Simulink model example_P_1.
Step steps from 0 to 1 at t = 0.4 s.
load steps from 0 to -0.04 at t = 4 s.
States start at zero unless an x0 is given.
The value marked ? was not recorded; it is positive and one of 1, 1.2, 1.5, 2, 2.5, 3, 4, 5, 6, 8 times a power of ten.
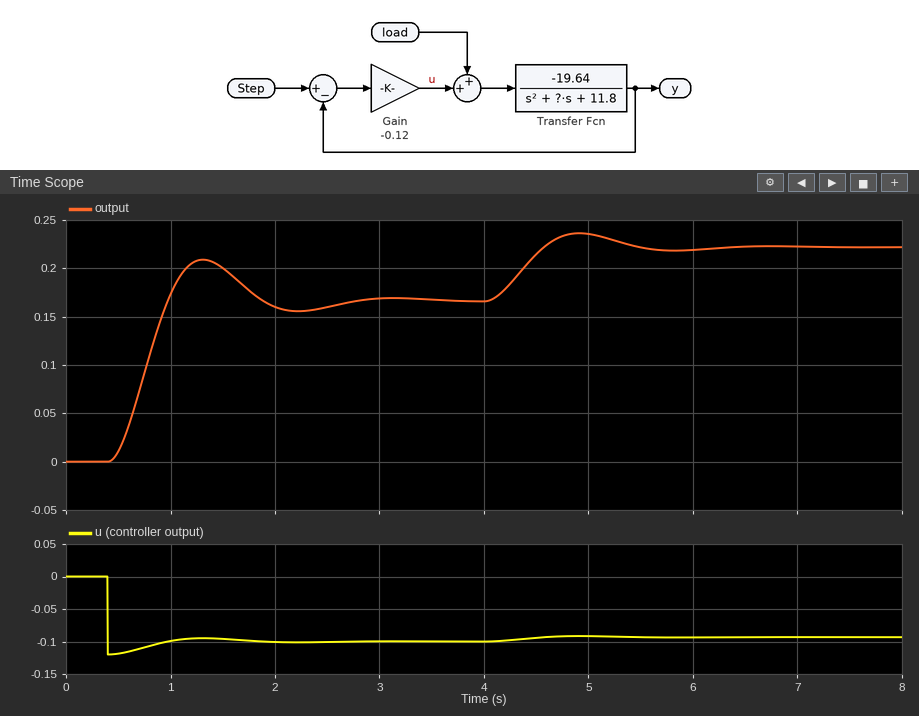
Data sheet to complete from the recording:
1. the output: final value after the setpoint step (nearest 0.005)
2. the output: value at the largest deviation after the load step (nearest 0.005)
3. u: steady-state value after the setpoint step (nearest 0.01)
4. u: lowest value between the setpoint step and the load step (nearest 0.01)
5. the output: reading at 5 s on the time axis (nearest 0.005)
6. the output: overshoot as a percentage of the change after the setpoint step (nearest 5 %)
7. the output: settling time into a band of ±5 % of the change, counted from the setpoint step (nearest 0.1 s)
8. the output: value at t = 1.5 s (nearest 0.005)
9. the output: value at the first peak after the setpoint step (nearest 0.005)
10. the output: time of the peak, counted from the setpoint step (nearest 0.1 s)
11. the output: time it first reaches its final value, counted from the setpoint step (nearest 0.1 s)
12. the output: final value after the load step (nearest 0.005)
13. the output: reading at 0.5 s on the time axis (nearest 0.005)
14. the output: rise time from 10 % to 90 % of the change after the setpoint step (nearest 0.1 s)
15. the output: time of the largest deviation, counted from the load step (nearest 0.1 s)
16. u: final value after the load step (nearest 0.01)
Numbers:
0.165
0.235
-0.10
-0.12
0.235
25 %
2.0 s
0.200
0.210
0.9 s
0.6 s
0.220
0.010
0.4 s
0.9 s
-0.09
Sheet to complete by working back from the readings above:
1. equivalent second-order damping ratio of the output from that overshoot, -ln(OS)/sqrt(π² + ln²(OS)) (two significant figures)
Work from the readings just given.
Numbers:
0.40
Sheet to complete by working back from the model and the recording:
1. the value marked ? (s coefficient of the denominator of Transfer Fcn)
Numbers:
3
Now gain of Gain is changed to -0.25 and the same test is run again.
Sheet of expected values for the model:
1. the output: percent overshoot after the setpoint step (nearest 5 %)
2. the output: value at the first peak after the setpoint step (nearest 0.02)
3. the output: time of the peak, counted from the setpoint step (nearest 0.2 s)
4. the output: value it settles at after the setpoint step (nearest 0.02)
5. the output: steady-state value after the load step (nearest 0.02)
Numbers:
30 %
0.38
0.8 s
0.30
0.34
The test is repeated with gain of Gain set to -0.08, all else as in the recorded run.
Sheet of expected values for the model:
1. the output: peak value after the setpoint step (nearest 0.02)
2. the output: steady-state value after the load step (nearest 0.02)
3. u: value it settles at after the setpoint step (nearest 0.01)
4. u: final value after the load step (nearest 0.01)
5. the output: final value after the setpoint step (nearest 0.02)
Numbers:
0.14
0.18
-0.07
-0.07
0.12
